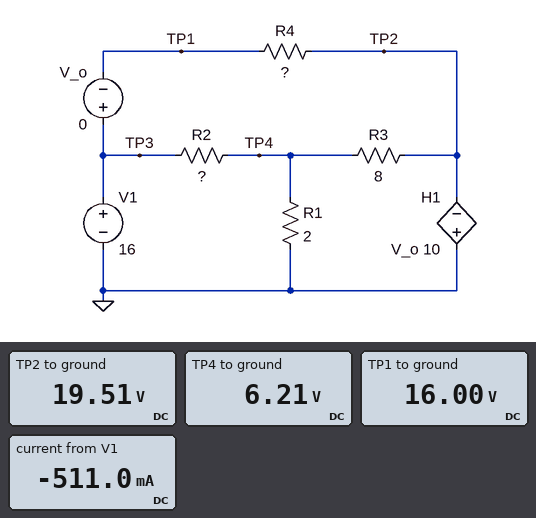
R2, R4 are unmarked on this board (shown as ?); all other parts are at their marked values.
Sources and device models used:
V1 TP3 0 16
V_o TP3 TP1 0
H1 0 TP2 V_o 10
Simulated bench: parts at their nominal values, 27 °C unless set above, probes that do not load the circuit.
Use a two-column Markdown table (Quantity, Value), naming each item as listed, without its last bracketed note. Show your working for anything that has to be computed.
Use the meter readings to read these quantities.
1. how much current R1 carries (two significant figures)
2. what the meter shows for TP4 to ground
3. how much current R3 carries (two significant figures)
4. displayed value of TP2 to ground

| Quantity | Value |
|---|---|
| how much current R1 carries | (6.21 V) / 2 Ω = 3.1 A |
| what the meter shows for TP4 to ground | 6.21 V |
| how much current R3 carries | (19.51 V - 6.21 V) / 8 Ω = 1.7 A |
| displayed value of TP2 to ground | 19.51 V |
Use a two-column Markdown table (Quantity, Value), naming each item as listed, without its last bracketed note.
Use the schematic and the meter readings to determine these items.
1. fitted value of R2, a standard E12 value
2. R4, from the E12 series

| Quantity | Value |
|---|---|
| fitted value of R2, a standard E12 value | 6.8 Ω |
| R4, from the E12 series | 1.8 Ω |
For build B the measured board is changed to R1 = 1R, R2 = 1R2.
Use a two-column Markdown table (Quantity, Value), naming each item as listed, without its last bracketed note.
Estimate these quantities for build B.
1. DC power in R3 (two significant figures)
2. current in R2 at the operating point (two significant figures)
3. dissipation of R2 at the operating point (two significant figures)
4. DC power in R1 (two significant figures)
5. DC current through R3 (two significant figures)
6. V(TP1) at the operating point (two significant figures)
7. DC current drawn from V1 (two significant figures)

| Quantity | Value |
|---|---|
| DC power in R3 | 16 W |
| current in R2 at the operating point | 6.6 A |
| dissipation of R2 at the operating point | 53 W |
| DC power in R1 | 65 W |
| DC current through R3 | 1.4 A |
| V(TP1) at the operating point | 16 V |
| DC current drawn from V1 | 4.7 A |
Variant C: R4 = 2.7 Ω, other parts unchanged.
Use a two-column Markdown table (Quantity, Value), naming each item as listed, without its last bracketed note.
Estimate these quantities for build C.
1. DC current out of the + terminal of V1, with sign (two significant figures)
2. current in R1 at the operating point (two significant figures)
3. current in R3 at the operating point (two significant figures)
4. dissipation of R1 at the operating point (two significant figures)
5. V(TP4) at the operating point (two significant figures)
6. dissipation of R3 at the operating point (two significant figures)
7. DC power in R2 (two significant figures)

| Quantity | Value |
|---|---|
| DC current out of the + terminal of V1, with sign | -810 mA |
| current in R1 at the operating point | 3.3 A |
| current in R3 at the operating point | 1.9 A |
| dissipation of R1 at the operating point | 22 W |
| V(TP4) at the operating point | 6.6 V |
| dissipation of R3 at the operating point | 29 W |
| DC power in R2 | 13 W |
